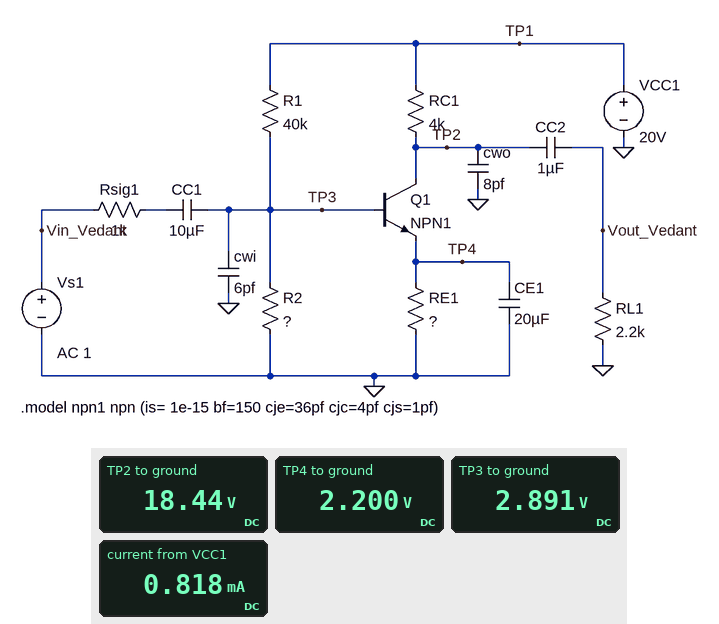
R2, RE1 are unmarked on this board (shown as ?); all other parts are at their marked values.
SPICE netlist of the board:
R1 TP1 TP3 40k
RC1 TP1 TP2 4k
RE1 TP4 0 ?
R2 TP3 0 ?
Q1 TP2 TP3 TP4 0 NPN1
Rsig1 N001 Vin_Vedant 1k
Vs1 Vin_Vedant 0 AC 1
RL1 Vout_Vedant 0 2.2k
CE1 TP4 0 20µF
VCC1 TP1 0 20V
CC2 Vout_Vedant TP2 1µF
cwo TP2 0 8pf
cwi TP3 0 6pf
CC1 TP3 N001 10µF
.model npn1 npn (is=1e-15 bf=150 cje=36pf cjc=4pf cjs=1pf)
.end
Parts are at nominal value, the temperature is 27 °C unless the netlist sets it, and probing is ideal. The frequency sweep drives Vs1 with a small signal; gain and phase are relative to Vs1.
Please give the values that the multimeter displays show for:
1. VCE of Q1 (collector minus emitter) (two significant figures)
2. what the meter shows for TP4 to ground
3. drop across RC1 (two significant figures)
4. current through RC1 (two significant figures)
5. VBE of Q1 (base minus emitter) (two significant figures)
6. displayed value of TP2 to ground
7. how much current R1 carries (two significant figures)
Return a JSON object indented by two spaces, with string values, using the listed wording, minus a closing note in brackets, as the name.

{
  "VCE of Q1 (collector minus emitter)": "16 V",
  "what the meter shows for TP4 to ground": "2.200 V",
  "drop across RC1": "1.6 V",
  "current through RC1": "390 µA",
  "VBE of Q1 (base minus emitter)": "690 mV",
  "displayed value of TP2 to ground": "18.44 V",
  "how much current R1 carries": "430 µA"
}
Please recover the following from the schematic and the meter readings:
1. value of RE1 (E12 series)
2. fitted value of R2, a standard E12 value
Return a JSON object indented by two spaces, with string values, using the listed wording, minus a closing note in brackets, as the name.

{
  "value of RE1": "5.6 kΩ",
  "fitted value of R2, a standard E12 value": "6.8 kΩ"
}
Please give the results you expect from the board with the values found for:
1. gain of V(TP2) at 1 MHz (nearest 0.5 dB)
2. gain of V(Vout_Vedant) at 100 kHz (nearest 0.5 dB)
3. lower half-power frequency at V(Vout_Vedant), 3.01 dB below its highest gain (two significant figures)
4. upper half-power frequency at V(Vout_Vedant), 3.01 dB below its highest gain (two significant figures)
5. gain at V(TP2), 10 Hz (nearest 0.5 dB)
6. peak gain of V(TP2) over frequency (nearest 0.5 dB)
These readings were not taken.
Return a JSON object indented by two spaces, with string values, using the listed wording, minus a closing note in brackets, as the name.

{
  "gain of V(TP2) at 1 MHz": "23.5 dB",
  "gain of V(Vout_Vedant) at 100 kHz": "24.5 dB",
  "lower half-power frequency at V(Vout_Vedant), 3.01 dB below its highest gain": "120 Hz",
  "upper half-power frequency at V(Vout_Vedant), 3.01 dB below its highest gain": "1.9 MHz",
  "gain at V(TP2), 10 Hz": "11.5 dB",
  "peak gain of V(TP2) over frequency": "24.5 dB"
}
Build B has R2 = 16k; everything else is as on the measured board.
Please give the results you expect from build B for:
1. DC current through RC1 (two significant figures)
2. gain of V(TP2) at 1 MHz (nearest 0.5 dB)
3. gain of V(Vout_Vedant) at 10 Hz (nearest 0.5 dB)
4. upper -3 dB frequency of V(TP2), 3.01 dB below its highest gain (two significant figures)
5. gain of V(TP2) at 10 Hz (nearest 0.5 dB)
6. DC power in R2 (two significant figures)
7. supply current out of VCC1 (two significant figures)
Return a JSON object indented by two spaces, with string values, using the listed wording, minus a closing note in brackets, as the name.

{
  "DC current through RC1": "880 µA",
  "gain of V(TP2) at 1 MHz": "29.5 dB",
  "gain of V(Vout_Vedant) at 10 Hz": "-4.5 dB",
  "upper -3 dB frequency of V(TP2), 3.01 dB below its highest gain": "1.3 MHz",
  "gain of V(TP2) at 10 Hz": "12.5 dB",
  "DC power in R2": "2.0 mW",
  "supply current out of VCC1": "1.2 mA"
}
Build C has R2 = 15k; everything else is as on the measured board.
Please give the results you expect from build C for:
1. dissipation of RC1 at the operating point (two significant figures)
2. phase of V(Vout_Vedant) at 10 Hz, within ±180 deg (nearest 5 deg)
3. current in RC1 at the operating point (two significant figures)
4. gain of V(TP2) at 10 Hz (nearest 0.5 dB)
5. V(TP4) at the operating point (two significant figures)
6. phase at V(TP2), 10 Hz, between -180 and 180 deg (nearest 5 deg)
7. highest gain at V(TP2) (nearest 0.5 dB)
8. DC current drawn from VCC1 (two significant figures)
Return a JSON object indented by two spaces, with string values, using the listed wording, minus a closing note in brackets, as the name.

{
  "dissipation of RC1 at the operating point": "2.8 mW",
  "phase of V(Vout_Vedant) at 10 Hz, within ±180 deg": "-25 deg",
  "current in RC1 at the operating point": "830 µA",
  "gain of V(TP2) at 10 Hz": "12.5 dB",
  "V(TP4) at the operating point": "4.7 V",
  "phase at V(TP2), 10 Hz, between -180 and 180 deg": "-105 deg",
  "highest gain at V(TP2)": "31.0 dB",
  "DC current drawn from VCC1": "1.2 mA"
}
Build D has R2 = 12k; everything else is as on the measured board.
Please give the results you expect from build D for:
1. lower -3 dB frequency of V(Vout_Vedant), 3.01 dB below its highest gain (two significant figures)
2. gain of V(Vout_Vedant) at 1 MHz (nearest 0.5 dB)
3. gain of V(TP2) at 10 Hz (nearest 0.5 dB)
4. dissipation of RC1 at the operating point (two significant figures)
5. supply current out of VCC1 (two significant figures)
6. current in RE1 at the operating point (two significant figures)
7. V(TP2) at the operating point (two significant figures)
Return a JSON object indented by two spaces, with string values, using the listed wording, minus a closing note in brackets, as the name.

{
  "lower -3 dB frequency of V(Vout_Vedant), 3.01 dB below its highest gain": "190 Hz",
  "gain of V(Vout_Vedant) at 1 MHz": "28.0 dB",
  "gain of V(TP2) at 10 Hz": "12.5 dB",
  "dissipation of RC1 at the operating point": "1.9 mW",
  "supply current out of VCC1": "1.1 mA",
  "current in RE1 at the operating point": "690 µA",
  "V(TP2) at the operating point": "17 V"
}
